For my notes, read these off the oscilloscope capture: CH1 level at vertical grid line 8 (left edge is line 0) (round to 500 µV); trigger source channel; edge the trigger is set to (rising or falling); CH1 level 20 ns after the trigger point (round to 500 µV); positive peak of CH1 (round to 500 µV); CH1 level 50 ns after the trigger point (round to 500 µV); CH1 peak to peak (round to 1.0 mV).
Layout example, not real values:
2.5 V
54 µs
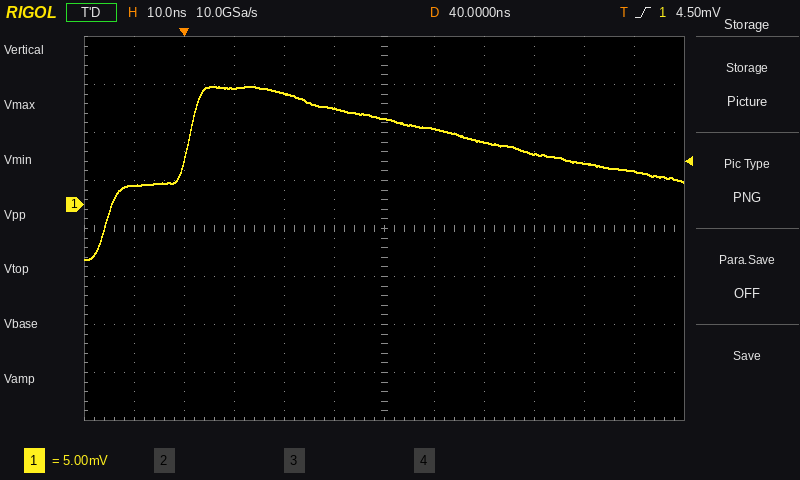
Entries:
6.5 mV
CH1
rising
11.5 mV
12.5 mV
8.0 mV
18.0 mV
